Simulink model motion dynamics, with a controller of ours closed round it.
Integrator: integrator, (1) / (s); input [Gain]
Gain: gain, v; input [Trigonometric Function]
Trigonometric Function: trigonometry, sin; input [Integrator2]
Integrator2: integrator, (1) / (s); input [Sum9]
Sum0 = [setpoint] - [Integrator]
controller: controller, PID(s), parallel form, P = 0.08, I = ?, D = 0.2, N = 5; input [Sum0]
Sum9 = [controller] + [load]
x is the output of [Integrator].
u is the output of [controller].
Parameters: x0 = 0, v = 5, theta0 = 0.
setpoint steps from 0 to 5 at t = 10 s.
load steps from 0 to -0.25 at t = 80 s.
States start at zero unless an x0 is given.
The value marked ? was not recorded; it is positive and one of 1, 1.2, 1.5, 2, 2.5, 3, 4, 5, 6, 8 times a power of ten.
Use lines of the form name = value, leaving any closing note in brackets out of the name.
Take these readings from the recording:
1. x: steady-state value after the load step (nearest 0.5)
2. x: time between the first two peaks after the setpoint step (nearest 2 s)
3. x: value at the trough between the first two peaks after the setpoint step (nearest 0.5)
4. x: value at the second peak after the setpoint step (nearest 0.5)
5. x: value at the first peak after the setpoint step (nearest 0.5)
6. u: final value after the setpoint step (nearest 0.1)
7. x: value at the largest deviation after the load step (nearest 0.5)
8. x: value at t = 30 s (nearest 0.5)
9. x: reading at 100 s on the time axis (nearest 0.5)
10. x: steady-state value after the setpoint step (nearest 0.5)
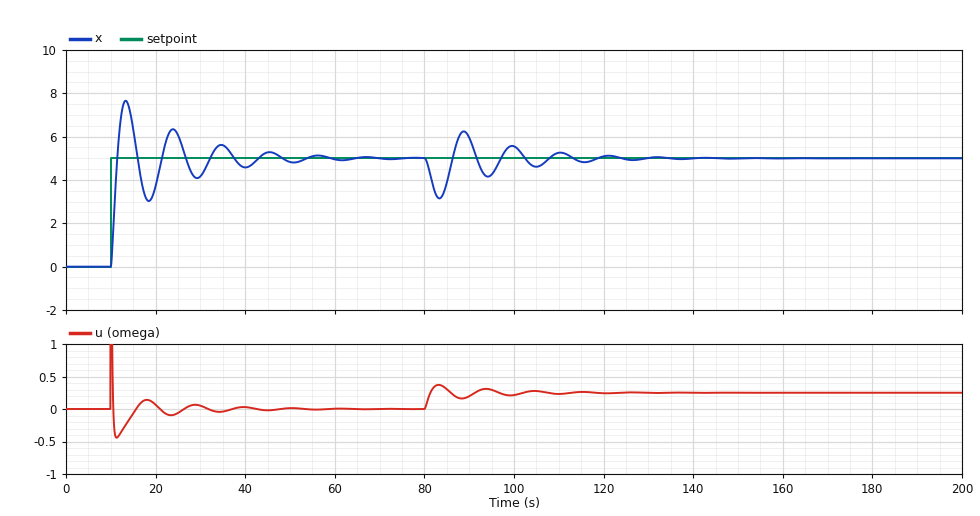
x: steady-state value after the load step = 5.0
x: time between the first two peaks after the setpoint step = 10 s
x: value at the trough between the first two peaks after the setpoint step = 3.0
x: value at the second peak after the setpoint step = 6.5
x: value at the first peak after the setpoint step = 7.5
u: final value after the setpoint step = 0.0
x: value at the largest deviation after the load step = 3.0
x: value at t = 30 s = 4.0
x: reading at 100 s on the time axis = 5.5
x: steady-state value after the setpoint step = 5.0
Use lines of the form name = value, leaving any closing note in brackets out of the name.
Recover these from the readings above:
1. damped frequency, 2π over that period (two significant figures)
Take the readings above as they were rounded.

damped frequency, 2π over that period = 0.63 rad/s
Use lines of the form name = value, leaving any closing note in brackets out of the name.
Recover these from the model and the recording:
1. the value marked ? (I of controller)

the value marked ? = 0.06
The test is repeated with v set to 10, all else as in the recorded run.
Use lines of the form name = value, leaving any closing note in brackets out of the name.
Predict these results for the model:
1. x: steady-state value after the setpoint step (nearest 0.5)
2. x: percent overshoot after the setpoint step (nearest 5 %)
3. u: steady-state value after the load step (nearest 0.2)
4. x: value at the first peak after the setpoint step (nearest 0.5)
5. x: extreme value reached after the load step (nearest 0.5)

x: steady-state value after the setpoint step = 5.0
x: percent overshoot after the setpoint step = 30 %
u: steady-state value after the load step = 0.2
x: value at the first peak after the setpoint step = 6.5
x: extreme value reached after the load step = 3.5
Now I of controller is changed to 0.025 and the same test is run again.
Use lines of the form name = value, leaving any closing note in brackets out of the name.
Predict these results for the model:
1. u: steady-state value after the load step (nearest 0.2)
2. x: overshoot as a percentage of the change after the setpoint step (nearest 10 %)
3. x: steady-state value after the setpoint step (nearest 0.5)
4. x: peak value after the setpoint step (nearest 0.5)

u: steady-state value after the load step = 0.2
x: overshoot as a percentage of the change after the setpoint step = 40 %
x: steady-state value after the setpoint step = 5.0
x: peak value after the setpoint step = 7.0
